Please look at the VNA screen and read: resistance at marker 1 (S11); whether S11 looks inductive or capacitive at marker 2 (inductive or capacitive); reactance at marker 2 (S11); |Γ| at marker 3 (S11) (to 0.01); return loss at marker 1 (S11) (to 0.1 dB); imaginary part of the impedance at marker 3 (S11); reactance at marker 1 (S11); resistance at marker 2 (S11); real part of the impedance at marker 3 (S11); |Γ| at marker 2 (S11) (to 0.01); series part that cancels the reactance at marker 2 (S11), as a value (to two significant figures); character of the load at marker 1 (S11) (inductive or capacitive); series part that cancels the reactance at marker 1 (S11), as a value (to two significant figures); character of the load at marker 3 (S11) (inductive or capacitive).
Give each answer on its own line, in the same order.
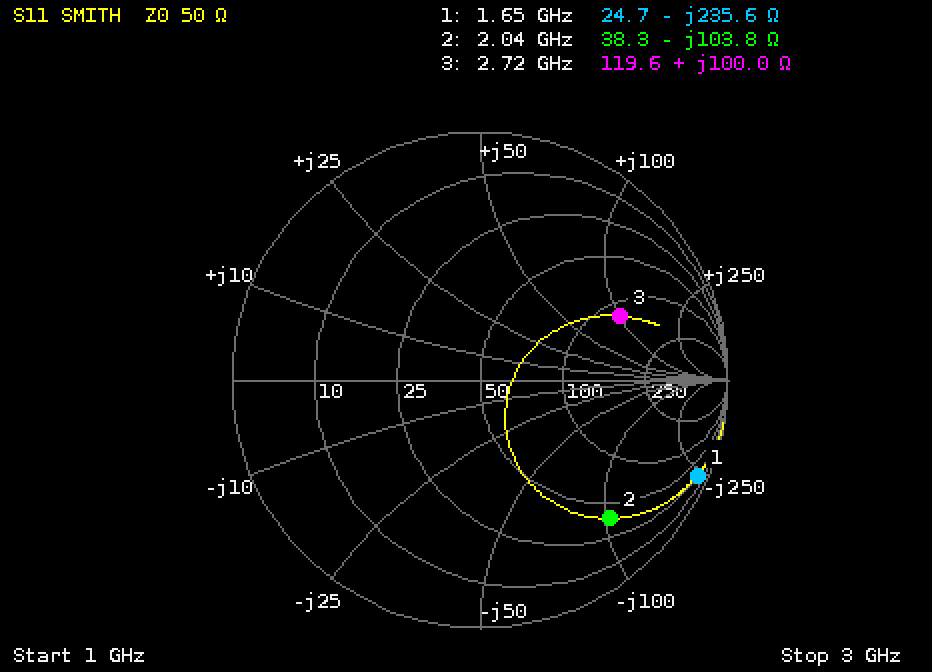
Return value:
24.7 Ω
capacitive
-103.8 Ω
0.62
0.4 dB
+100.0 Ω
-235.6 Ω
38.3 Ω
119.6 Ω
0.77
8.1 nH
capacitive
23 nH
inductive
